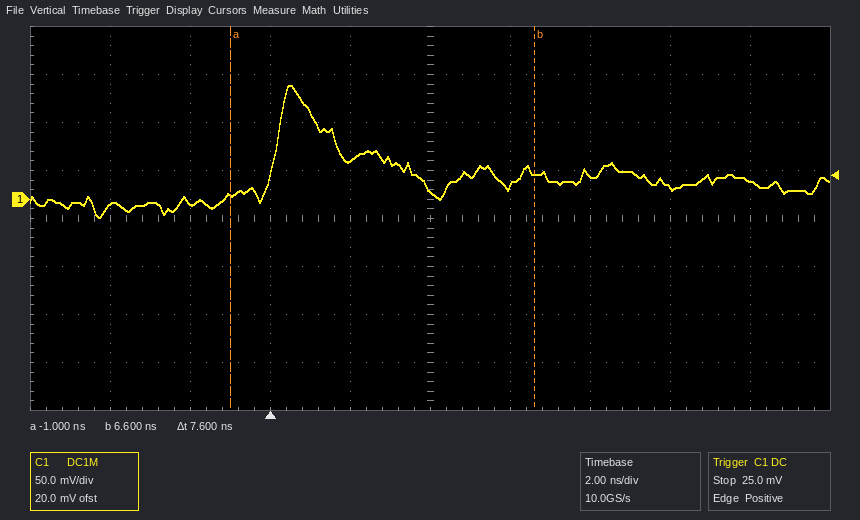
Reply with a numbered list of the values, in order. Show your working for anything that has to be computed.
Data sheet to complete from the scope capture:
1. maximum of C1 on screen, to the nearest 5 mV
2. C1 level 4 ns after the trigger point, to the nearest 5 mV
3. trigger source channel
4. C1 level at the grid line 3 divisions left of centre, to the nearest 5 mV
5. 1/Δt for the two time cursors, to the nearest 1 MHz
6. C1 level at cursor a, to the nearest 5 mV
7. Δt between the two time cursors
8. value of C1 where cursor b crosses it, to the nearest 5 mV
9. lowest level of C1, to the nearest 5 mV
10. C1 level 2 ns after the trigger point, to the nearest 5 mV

1. 120 mV
2. 10 mV
3. C1
4. -5 mV
5. 1 / 7.6 ns ≈ 132 MHz
6. 5 mV
7. 7.6 ns
8. 25 mV
9. -20 mV
10. 40 mV
